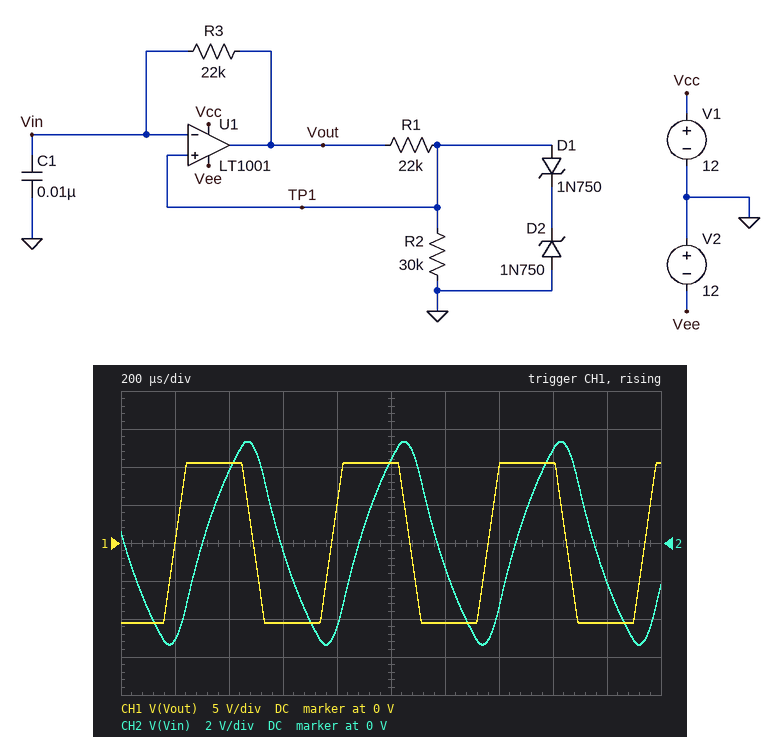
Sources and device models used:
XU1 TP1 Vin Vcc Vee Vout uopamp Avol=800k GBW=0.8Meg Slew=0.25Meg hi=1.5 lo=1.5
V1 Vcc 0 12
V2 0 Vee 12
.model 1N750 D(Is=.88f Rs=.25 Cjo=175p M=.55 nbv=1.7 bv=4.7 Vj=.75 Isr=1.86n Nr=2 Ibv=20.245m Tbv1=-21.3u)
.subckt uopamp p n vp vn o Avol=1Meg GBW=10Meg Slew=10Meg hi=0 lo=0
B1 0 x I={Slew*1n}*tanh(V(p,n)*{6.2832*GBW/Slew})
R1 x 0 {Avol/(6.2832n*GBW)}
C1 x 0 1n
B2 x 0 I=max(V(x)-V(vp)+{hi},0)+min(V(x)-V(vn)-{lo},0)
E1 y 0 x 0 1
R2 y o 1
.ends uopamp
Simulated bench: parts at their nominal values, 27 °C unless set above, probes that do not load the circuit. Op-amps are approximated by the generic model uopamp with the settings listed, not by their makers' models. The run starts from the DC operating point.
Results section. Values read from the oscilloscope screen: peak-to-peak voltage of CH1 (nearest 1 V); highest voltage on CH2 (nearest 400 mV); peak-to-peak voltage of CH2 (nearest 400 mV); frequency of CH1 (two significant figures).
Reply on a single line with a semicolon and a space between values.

21 V; 5.2 V; 10.8 V; 1.7 kHz
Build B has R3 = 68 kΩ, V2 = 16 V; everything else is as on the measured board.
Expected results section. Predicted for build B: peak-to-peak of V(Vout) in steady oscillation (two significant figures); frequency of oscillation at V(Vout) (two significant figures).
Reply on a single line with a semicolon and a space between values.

25 V; 730 Hz
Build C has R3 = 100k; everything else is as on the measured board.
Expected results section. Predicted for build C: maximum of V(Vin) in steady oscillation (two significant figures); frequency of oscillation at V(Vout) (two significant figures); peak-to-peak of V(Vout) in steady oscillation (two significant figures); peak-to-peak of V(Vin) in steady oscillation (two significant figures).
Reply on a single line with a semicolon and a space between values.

5.1 V; 450 Hz; 21 V; 10 V
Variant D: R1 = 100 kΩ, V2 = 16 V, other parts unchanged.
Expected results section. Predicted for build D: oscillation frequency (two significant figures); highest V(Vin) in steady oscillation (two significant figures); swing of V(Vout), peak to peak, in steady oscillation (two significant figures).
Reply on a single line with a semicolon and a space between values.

2.7 kHz; 3.0 V; 25 V
